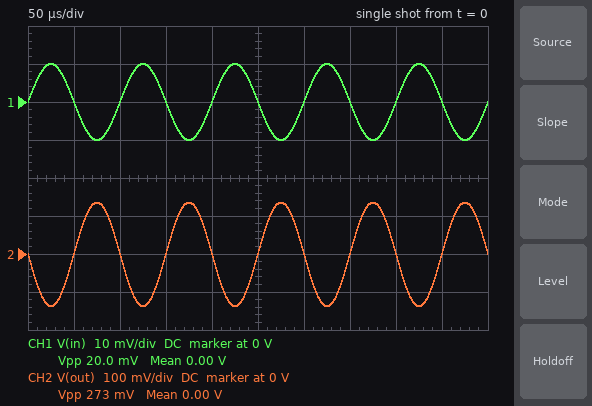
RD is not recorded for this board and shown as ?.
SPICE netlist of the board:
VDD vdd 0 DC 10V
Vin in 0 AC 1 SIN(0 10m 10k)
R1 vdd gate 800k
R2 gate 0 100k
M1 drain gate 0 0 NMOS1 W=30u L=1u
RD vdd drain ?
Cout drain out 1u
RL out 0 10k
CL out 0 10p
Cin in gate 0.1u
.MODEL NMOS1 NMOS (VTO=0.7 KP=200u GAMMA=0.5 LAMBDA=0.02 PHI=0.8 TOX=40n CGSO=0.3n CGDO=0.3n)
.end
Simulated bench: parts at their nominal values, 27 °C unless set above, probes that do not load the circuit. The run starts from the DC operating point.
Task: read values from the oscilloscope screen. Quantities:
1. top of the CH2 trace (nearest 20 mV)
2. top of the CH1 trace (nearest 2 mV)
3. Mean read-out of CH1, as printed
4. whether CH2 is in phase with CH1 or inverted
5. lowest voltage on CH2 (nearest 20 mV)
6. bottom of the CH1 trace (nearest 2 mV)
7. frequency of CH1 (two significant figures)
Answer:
140 mV
10 mV
0.00 V
inverted
-140 mV
-10 mV
10 kHz
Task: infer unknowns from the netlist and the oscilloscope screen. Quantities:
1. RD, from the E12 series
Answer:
12 kΩ
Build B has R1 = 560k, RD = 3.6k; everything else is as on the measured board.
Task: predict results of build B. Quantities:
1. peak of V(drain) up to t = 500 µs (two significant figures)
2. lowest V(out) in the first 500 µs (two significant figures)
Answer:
2.6 V
-120 mV
